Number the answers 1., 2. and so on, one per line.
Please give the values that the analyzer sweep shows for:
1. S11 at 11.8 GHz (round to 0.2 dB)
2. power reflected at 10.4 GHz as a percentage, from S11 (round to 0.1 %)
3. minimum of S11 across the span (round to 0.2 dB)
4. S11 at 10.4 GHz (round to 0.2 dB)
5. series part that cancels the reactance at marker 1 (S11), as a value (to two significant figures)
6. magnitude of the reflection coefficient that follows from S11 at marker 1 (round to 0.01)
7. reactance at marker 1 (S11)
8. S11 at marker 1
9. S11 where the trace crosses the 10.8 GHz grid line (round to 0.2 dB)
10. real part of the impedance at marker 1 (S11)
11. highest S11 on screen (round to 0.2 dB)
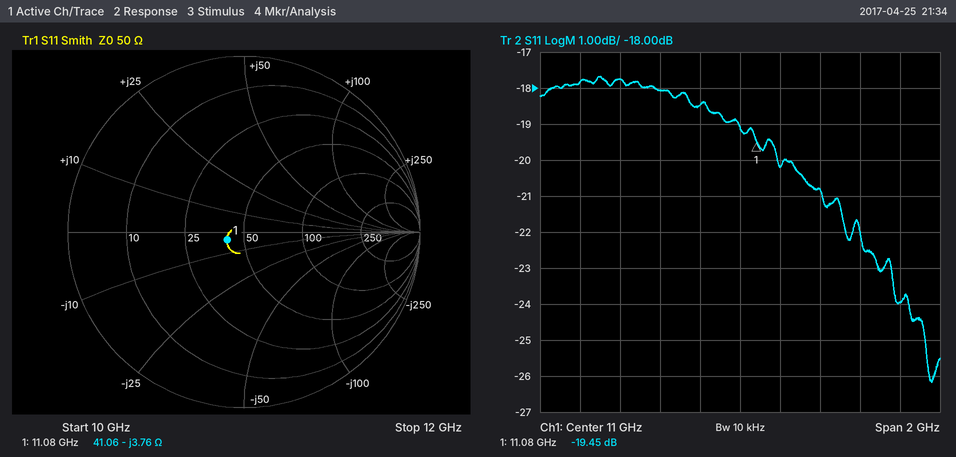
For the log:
1. -24.0 dB
2. 1.7 %
3. -26.2 dB
4. -17.8 dB
5. 54 pH
6. 0.11
7. -3.76 Ω
8. -19.45 dB
9. -18.4 dB
10. 41.06 Ω
11. -17.6 dB
